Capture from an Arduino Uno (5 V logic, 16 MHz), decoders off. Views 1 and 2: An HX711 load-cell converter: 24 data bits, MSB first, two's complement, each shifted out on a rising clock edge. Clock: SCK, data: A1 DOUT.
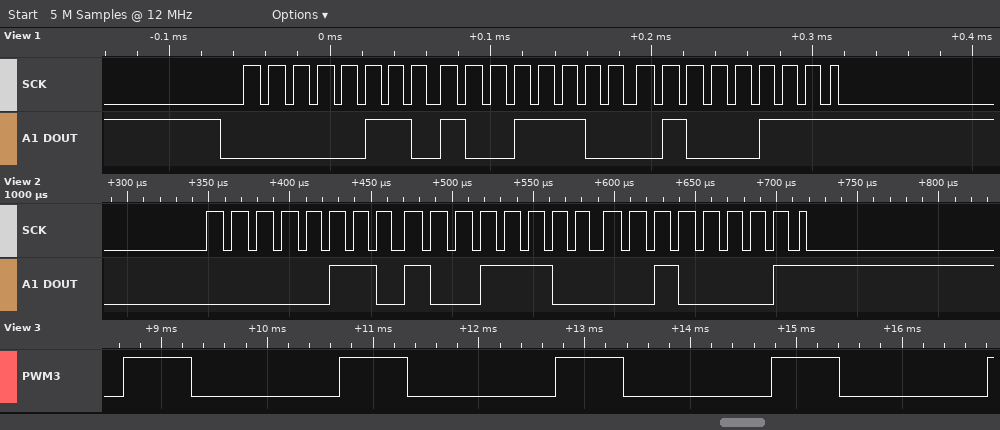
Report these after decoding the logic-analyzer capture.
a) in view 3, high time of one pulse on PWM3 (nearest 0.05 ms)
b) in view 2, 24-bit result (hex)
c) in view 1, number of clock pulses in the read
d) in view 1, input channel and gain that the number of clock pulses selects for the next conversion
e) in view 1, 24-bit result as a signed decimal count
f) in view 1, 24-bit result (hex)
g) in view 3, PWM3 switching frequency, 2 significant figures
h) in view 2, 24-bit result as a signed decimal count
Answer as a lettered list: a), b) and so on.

a) 0.65 ms
b) 0x069C21
c) 25
d) channel A, gain 128
e) 433223
f) 0x069C47
g) 490 Hz
h) 433185
